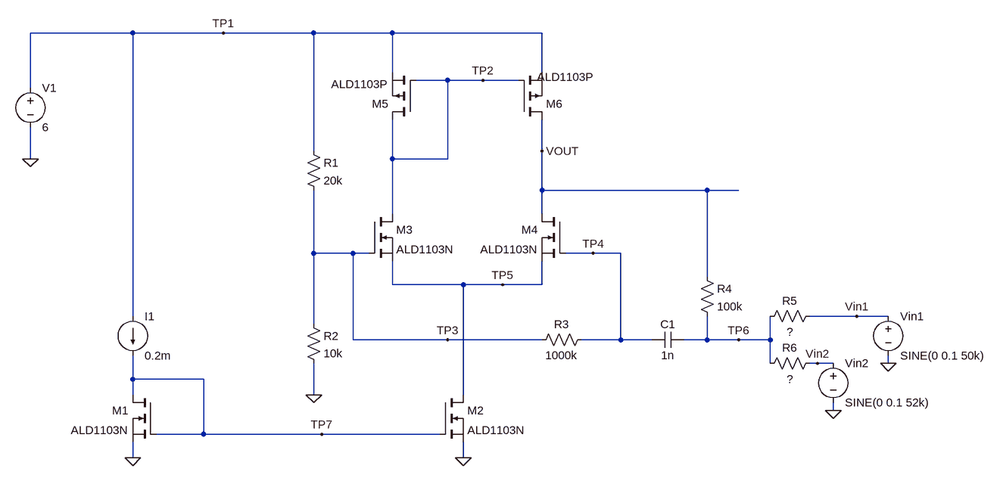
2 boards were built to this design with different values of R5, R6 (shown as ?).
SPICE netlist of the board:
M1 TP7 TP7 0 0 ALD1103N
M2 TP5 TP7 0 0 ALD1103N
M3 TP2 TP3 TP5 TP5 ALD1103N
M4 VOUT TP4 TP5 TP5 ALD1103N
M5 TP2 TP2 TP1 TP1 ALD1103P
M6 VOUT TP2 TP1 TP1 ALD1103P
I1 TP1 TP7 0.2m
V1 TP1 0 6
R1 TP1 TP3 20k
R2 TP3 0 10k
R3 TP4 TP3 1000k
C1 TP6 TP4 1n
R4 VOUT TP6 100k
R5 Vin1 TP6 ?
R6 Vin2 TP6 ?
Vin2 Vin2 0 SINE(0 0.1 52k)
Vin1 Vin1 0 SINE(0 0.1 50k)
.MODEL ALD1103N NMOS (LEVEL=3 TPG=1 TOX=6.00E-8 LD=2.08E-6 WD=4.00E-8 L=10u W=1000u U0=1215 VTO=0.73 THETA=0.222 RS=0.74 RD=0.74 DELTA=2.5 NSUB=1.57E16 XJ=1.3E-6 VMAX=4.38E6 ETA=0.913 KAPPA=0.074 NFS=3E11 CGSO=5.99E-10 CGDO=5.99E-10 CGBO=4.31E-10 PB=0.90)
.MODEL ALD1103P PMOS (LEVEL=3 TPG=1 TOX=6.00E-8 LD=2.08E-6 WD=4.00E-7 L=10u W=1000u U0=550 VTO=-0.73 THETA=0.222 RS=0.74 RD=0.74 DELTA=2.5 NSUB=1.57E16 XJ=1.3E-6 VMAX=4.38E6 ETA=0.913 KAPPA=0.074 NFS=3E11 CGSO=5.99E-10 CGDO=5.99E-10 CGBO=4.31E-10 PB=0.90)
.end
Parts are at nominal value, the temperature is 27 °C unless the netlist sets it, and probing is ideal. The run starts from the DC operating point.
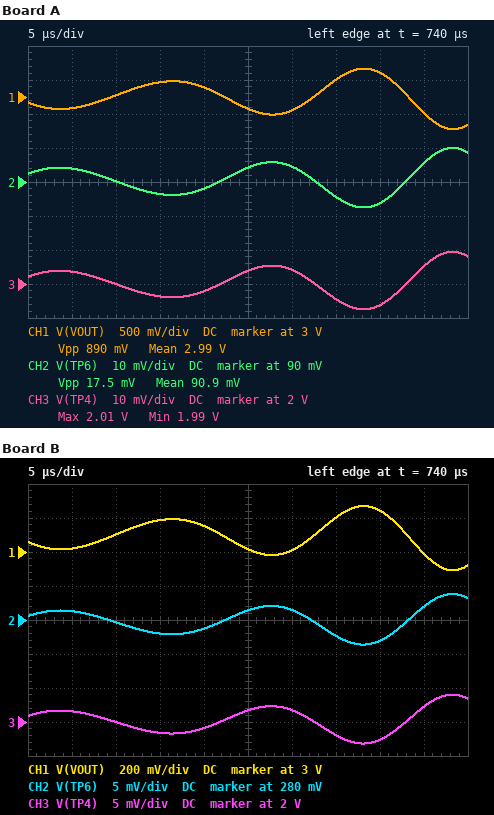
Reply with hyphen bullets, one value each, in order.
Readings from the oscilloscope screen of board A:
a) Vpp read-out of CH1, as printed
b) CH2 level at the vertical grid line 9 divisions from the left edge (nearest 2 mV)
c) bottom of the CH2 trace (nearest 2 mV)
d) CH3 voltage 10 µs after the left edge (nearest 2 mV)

- 890 mV
- 96 mV
- 82 mV
- 2.000 V
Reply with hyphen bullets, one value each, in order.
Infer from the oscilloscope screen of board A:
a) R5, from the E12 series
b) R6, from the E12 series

- 5.6 kΩ
- 6.8 kΩ
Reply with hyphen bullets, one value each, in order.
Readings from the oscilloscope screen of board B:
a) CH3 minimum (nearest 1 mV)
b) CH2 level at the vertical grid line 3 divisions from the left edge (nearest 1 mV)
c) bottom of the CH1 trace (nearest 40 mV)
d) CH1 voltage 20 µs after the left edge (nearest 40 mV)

- 1.997 V
- 278 mV
- 2.88 V
- 3.16 V
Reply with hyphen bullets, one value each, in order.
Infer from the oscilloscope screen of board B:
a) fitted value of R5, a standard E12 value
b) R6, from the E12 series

- 18 kΩ
- 22 kΩ
